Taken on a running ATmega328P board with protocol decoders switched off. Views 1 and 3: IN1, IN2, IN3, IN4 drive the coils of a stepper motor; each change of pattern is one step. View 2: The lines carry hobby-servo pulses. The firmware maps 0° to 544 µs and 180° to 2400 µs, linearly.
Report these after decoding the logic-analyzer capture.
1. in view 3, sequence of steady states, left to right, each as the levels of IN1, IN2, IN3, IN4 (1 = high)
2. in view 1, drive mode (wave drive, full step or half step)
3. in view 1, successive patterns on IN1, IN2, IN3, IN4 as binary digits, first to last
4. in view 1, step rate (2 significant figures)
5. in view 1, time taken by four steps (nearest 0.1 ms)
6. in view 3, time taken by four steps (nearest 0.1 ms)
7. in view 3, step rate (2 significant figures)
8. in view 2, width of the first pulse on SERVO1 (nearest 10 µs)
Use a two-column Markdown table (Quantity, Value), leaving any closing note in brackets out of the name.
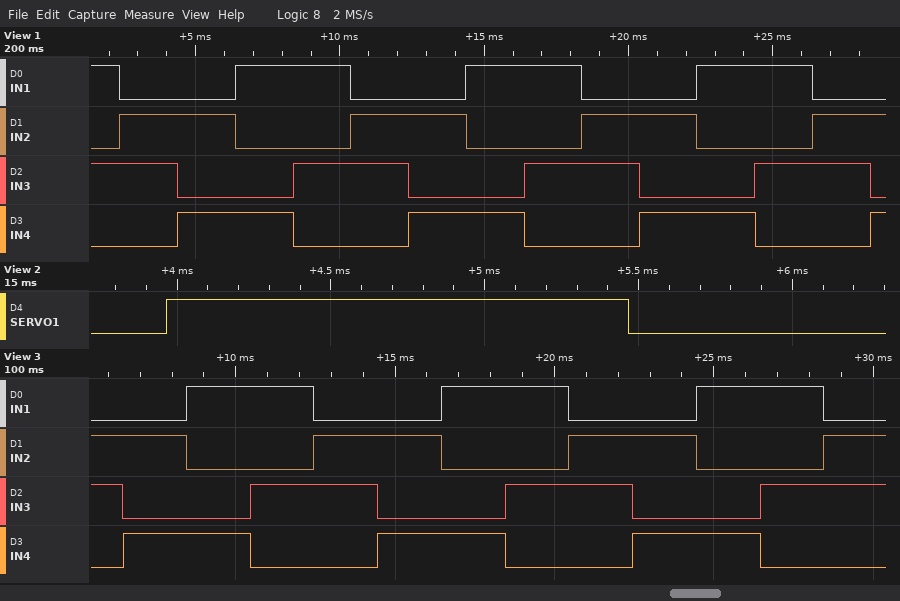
| Quantity | Value |
|---|---|
| in view 3, sequence of steady states, left to right, each as the levels of IN1, IN2, IN3, IN4 | 0110 0101 1001 1010 0110 0101 1001 1010 0110 0101 1001 1010 0110 |
| in view 1, drive mode | full step |
| in view 1, successive patterns on IN1, IN2, IN3, IN4 as binary digits, first to last | 1010 0110 0101 1001 1010 0110 0101 1001 1010 0110 0101 1001 1010 0110 0101 |
| in view 1, step rate | 500 steps/s |
| in view 1, time taken by four steps | 8.0 ms |
| in view 3, time taken by four steps | 8.0 ms |
| in view 3, step rate | 500 steps/s |
| in view 2, width of the first pulse on SERVO1 | 1500 µs |
